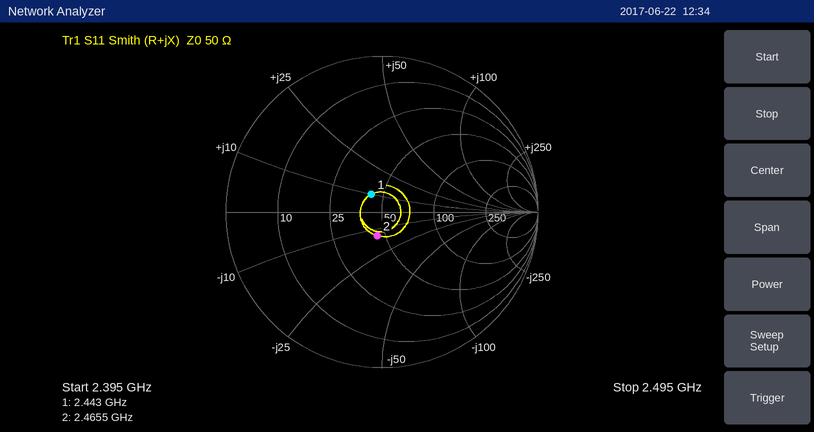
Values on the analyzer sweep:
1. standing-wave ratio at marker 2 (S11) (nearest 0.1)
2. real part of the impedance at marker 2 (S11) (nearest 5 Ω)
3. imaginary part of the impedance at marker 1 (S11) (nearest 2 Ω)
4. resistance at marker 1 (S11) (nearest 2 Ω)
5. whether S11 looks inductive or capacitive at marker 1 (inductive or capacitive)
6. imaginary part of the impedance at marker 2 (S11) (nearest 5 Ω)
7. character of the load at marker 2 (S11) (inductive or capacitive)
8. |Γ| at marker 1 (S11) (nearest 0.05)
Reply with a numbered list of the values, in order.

1. 1.4
2. 45 Ω
3. +10 Ω
4. 42 Ω
5. inductive
6. -15 Ω
7. capacitive
8. 0.15
